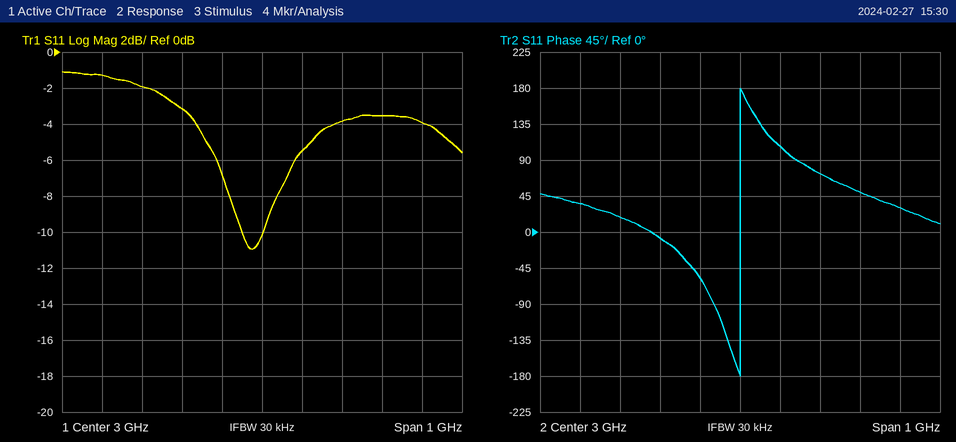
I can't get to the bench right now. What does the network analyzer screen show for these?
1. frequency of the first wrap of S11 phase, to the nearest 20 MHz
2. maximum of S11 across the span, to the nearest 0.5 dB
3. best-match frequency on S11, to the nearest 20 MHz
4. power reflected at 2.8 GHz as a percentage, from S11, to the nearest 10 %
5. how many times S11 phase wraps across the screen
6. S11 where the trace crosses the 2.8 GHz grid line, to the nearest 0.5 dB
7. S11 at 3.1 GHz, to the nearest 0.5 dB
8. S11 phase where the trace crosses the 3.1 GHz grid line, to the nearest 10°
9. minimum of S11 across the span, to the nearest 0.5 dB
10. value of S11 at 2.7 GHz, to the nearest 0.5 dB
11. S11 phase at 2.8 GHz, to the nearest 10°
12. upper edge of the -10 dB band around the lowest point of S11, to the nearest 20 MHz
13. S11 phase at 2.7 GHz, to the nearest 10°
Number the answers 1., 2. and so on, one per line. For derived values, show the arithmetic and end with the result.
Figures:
1. 3.00 GHz
2. -1.0 dB
3. 2.98 GHz
4. 10^(-3/10) ≈ 50 %
5. 1
6. -3.0 dB
7. -5.5 dB
8. 110°
9. -11.0 dB
10. -2.0 dB
11. -10°
12. 3.00 GHz
13. 20°
